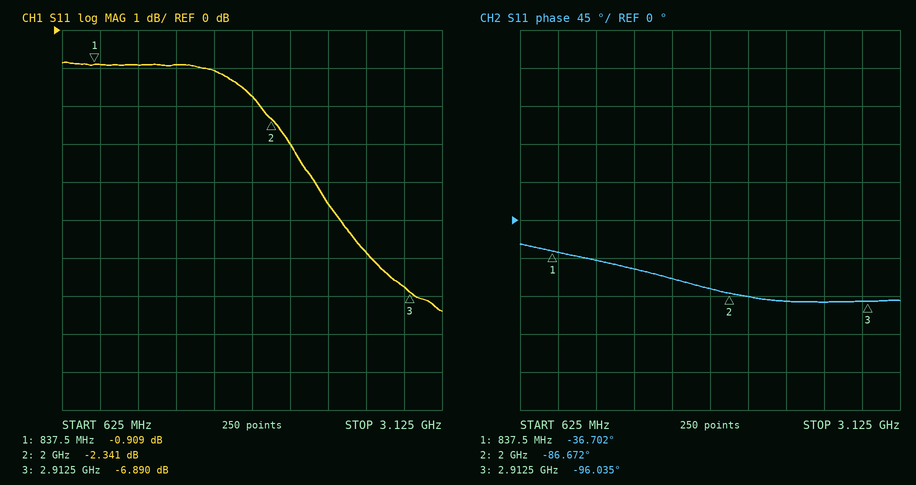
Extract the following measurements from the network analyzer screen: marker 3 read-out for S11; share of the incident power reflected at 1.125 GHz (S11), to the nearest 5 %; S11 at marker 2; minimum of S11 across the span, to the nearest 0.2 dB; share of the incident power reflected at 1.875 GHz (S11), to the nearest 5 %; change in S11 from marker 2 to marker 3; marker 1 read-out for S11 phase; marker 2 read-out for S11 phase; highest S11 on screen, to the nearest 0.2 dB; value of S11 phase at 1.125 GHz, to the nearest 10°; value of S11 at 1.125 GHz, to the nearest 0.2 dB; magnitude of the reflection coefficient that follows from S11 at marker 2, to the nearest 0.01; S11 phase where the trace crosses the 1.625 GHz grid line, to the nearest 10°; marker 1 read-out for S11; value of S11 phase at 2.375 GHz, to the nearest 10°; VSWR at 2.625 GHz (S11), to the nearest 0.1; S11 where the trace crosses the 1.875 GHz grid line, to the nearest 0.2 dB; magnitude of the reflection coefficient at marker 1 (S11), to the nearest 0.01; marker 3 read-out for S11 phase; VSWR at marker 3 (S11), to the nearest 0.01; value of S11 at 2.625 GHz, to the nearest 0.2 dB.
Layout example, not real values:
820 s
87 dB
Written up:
-6.890 dB
80 %
-2.341 dB
-7.4 dB
65 %
-4.549 dB
-36.702°
-86.672°
-0.8 dB
-50°
-1.0 dB
0.76
-70°
-0.909 dB
-100°
3.1
-1.8 dB
0.90
-96.035°
2.65
-5.8 dB
